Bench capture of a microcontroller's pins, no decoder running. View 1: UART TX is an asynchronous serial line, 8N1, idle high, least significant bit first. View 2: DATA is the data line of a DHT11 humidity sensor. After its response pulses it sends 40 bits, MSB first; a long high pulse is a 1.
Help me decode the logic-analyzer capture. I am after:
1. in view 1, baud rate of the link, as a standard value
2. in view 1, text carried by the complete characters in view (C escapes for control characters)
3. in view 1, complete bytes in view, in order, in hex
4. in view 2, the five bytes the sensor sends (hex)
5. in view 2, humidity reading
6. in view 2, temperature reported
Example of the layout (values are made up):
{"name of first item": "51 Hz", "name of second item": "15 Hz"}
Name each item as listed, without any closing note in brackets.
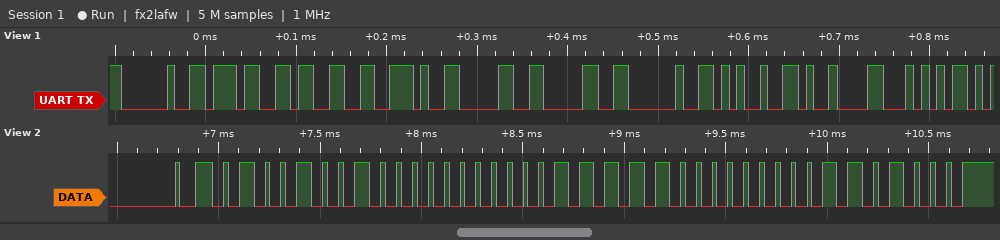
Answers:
{"in view 1, baud rate of the link, as a standard value": "115200 baud", "in view 1, text carried by the complete characters in view": "\" 73.00 %\\tT\"", "in view 1, complete bytes in view, in order, in hex": "0x20 0x37 0x33 0x2E 0x30 0x30 0x20 0x25 0x09 0x54", "in view 2, the five bytes the sensor sends": "49 00 1F 00 68", "in view 2, humidity reading": "73 %", "in view 2, temperature reported": "31.0 °C"}
